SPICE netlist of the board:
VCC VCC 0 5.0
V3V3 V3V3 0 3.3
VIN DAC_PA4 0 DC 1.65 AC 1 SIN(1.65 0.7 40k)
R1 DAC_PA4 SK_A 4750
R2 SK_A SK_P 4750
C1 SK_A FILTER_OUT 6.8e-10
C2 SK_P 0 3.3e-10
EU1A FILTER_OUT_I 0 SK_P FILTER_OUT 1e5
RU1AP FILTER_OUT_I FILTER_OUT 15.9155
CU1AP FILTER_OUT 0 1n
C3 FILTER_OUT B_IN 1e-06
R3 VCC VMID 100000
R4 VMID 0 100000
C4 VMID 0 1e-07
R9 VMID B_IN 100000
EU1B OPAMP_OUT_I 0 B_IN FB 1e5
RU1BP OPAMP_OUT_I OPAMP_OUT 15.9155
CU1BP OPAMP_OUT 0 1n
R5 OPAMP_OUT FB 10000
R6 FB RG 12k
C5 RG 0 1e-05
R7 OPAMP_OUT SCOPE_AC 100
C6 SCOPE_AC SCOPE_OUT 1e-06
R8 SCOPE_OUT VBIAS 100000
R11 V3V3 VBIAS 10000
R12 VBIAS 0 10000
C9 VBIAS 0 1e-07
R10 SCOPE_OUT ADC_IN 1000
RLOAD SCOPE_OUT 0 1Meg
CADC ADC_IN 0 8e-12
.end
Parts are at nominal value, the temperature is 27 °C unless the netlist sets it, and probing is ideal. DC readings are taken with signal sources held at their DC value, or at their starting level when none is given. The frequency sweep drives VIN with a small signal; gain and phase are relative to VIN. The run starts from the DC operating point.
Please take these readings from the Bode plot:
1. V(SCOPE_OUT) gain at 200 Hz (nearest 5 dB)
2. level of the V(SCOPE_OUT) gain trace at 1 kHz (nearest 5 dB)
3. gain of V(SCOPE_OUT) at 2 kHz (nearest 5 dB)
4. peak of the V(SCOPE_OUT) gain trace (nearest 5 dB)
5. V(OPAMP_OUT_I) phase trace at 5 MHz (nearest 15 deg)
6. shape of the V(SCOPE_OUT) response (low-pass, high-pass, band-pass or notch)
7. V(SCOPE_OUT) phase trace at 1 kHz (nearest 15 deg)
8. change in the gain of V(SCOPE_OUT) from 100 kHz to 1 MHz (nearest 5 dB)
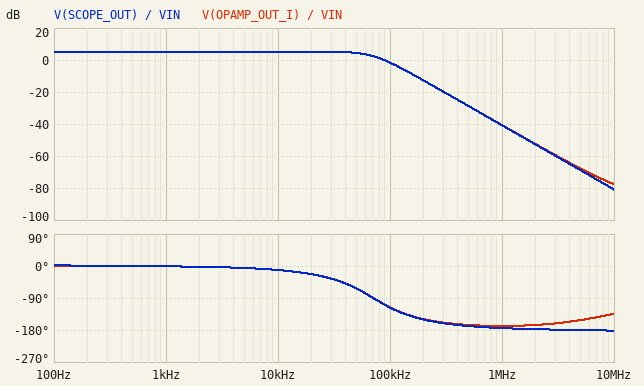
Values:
5 dB
5 dB
5 dB
5 dB
-150 deg
low-pass
0 deg
-40 dB
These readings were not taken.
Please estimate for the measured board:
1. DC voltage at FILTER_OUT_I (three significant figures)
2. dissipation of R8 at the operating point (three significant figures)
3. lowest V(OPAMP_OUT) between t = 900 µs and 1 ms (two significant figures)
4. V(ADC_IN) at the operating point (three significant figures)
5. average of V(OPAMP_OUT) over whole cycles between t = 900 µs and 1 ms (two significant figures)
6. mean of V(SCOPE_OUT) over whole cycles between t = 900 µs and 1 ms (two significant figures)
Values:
1.65 V
223 nW
1.3 V
1.49 V
2.5 V
1.5 V
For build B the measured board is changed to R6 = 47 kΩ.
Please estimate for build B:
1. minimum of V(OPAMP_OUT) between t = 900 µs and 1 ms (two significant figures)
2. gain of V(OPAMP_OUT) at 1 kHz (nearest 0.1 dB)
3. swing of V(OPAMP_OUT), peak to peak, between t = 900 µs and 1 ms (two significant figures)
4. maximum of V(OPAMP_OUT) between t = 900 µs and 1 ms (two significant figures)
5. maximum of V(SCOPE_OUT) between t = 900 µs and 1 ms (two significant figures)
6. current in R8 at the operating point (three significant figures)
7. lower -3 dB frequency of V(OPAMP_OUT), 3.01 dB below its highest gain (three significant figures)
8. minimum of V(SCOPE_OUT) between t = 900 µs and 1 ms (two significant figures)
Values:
1.7 V
1.7 dB
1.6 V
3.3 V
2.3 V
1.49 µA
1.11 Hz
680 mV
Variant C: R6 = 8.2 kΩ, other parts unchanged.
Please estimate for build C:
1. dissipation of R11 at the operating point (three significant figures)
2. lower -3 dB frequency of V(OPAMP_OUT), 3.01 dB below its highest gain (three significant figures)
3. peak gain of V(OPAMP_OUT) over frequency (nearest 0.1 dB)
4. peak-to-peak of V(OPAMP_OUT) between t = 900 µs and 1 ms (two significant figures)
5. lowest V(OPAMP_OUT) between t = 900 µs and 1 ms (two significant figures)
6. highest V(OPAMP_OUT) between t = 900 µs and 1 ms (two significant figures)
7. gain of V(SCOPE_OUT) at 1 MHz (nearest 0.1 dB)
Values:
275 µW
2.12 Hz
6.9 dB
3.0 V
1.0 V
4.0 V
-39.1 dB
